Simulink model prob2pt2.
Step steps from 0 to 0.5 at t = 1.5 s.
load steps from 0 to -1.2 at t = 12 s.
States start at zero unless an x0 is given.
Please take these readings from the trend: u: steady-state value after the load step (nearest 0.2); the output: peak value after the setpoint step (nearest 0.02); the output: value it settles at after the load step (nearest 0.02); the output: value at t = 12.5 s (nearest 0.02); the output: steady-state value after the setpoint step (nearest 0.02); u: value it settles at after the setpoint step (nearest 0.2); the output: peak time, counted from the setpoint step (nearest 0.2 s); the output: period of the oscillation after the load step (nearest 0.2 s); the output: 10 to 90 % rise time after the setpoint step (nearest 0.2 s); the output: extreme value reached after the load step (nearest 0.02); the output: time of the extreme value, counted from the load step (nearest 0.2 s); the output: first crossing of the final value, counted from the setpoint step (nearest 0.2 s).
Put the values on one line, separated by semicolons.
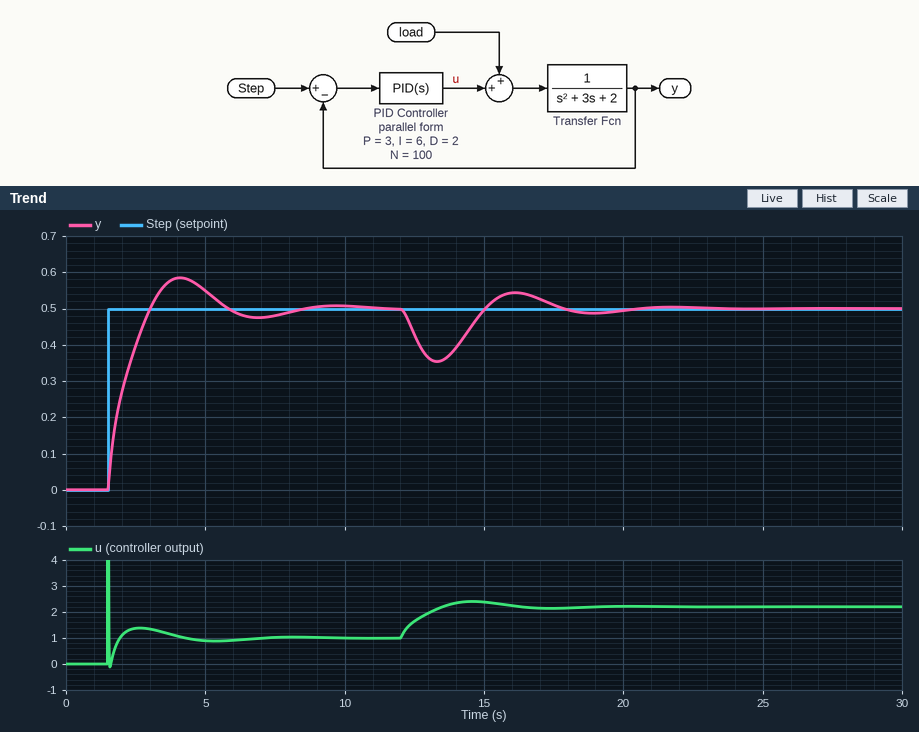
2.2; 0.58; 0.50; 0.42; 0.50; 1.0; 2.6 s; 5.6 s; 1.2 s; 0.36; 1.4 s; 1.6 s
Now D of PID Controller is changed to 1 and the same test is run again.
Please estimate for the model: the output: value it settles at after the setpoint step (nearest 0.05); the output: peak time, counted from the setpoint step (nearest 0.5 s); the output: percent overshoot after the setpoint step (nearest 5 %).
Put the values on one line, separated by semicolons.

0.50; 2.0 s; 25 %
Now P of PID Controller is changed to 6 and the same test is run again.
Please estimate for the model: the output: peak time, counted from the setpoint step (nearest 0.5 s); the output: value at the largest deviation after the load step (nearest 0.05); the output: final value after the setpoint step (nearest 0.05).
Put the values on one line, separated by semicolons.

2.0 s; 0.40; 0.50
